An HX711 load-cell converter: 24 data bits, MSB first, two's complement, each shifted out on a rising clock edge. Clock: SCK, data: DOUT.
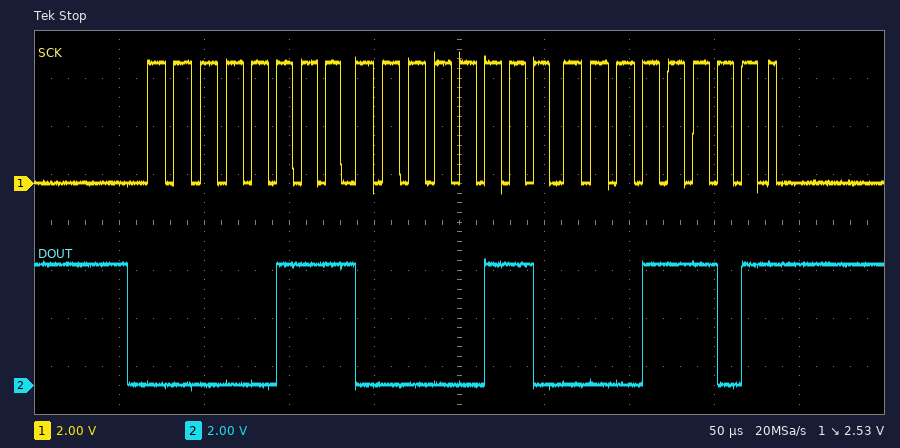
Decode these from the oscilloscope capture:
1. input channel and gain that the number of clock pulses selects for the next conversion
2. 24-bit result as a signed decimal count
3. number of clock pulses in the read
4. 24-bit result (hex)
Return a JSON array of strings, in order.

["channel A, gain 128", "460317", "25", "0x07061D"]
